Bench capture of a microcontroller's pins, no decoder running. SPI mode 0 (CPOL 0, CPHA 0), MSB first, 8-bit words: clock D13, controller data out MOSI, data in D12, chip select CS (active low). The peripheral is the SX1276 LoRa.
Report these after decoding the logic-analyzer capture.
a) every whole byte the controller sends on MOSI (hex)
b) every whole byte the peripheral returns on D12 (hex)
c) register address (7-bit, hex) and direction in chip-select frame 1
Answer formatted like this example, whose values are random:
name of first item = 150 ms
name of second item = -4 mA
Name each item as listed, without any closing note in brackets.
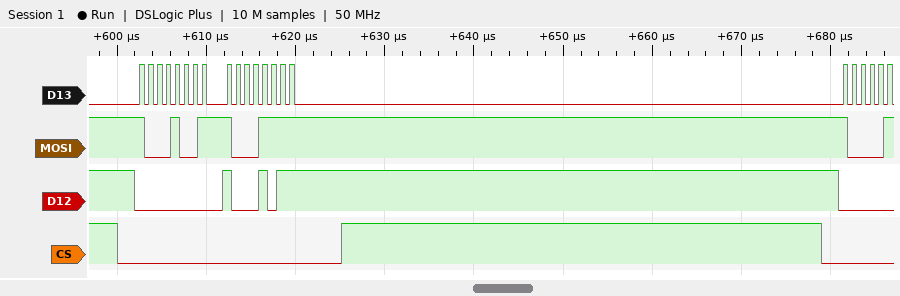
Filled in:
every whole byte the controller sends on MOSI = 0x89 0x8F
every whole byte the peripheral returns on D12 = 0x00 0x8B
register address (7-bit, hex) and direction in chip-select frame 1 = 0x09 write
